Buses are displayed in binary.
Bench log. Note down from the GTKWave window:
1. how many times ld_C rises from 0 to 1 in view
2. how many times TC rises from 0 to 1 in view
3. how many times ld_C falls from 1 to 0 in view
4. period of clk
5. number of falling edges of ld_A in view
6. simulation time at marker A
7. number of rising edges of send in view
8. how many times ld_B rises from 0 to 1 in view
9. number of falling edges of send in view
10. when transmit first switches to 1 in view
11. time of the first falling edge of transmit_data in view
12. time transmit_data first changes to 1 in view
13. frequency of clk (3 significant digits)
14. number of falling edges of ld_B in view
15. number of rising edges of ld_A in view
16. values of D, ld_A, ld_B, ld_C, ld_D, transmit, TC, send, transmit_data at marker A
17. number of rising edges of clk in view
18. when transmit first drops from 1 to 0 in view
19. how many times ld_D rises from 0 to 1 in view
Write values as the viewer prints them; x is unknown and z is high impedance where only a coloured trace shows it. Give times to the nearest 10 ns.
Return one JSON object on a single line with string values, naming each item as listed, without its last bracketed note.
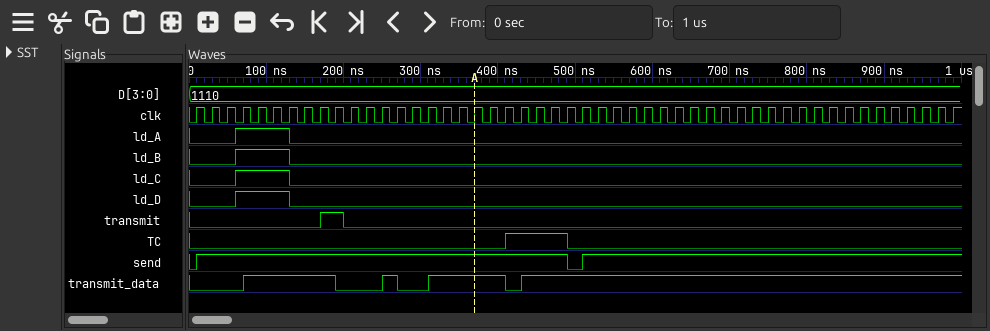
{"how many times ld_C rises from 0 to 1 in view": "1", "how many times TC rises from 0 to 1 in view": "1", "how many times ld_C falls from 1 to 0 in view": "1", "period of clk": "20 ns", "number of falling edges of ld_A in view": "1", "simulation time at marker A": "370 ns", "number of rising edges of send in view": "2", "how many times ld_B rises from 0 to 1 in view": "1", "number of falling edges of send in view": "1", "when transmit first switches to 1 in view": "170 ns", "time of the first falling edge of transmit_data in view": "190 ns", "time transmit_data first changes to 1 in view": "70 ns", "frequency of clk": "50.0 MHz", "number of falling edges of ld_B in view": "1", "number of rising edges of ld_A in view": "1", "values of D, ld_A, ld_B, ld_C, ld_D, transmit, TC, send, transmit_data at marker A": "D=1110, ld_A=0, ld_B=0, ld_C=0, ld_D=0, transmit=0, TC=0, send=1, transmit_data=1", "number of rising edges of clk in view": "50", "when transmit first drops from 1 to 0 in view": "200 ns", "how many times ld_D rises from 0 to 1 in view": "1"}
